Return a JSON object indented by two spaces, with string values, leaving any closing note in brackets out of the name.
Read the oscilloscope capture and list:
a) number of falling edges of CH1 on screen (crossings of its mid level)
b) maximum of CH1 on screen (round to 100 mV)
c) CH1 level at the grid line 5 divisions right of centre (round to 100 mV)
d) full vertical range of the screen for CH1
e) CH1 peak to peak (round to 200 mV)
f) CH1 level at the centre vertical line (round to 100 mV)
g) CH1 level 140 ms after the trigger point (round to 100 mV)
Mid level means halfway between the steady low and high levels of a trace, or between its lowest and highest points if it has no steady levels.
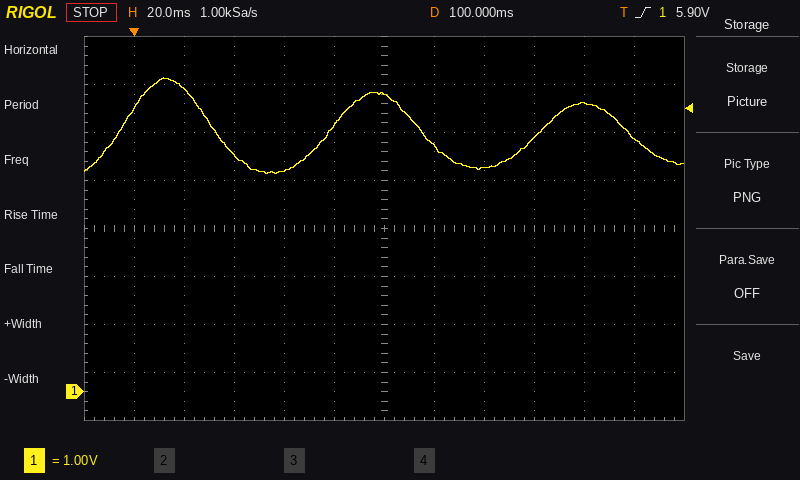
{
  "number of falling edges of CH1 on screen": "3",
  "maximum of CH1 on screen": "6.5 V",
  "CH1 level at the grid line 5 divisions right of centre": "5.3 V",
  "full vertical range of the screen for CH1": "8 V",
  "CH1 peak to peak": "2.0 V",
  "CH1 level at the centre vertical line": "6.2 V",
  "CH1 level 140 ms after the trigger point": "4.7 V"
}
